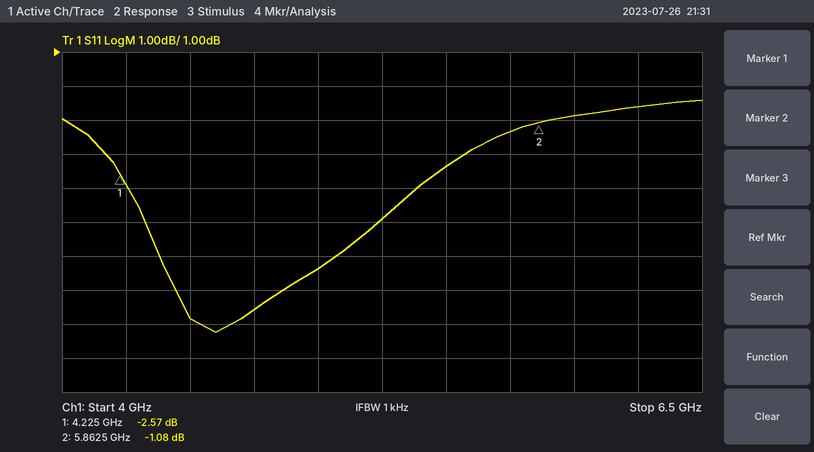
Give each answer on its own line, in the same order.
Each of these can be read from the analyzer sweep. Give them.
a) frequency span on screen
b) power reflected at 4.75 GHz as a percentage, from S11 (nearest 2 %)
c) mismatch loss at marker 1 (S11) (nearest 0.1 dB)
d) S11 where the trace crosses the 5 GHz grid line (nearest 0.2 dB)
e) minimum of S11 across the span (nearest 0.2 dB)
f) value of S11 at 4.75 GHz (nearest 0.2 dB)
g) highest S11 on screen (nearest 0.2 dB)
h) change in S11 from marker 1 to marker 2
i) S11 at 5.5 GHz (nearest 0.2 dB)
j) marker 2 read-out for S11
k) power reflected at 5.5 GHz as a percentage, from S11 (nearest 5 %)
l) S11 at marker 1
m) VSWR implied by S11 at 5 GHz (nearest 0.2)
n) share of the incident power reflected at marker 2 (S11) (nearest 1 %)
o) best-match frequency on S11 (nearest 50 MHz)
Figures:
2.5 GHz
22 %
3.5 dB
-5.4 dB
-7.2 dB
-6.6 dB
-0.4 dB
1.49 dB
-2.4 dB
-1.08 dB
60 %
-2.57 dB
3.4
78 %
4.60 GHz
